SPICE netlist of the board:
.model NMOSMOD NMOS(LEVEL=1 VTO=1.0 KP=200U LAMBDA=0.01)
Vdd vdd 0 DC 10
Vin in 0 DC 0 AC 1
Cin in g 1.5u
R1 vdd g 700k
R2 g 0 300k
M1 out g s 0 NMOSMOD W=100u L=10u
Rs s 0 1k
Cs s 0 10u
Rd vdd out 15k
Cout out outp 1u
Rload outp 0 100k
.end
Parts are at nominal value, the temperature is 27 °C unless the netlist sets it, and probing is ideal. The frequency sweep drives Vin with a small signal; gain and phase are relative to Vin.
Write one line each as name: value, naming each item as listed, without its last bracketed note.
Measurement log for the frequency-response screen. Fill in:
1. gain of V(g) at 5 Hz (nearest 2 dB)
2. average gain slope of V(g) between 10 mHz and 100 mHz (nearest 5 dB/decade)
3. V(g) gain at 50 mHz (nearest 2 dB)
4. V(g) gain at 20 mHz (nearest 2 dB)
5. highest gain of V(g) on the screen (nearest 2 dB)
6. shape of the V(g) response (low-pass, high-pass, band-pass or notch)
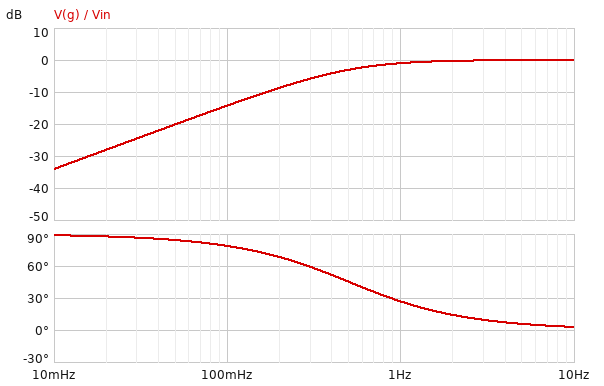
gain of V(g) at 5 Hz: 0 dB
average gain slope of V(g) between 10 mHz and 100 mHz: 20 dB/decade
V(g) gain at 50 mHz: -20 dB
V(g) gain at 20 mHz: -28 dB
highest gain of V(g) on the screen: 0 dB
shape of the V(g) response: high-pass
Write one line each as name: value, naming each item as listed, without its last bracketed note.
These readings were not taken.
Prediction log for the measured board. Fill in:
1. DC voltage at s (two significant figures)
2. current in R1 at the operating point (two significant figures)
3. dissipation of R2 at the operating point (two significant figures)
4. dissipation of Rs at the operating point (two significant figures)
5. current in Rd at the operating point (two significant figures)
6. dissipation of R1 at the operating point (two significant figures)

DC voltage at s: 610 mV
current in R1 at the operating point: 10 µA
dissipation of R2 at the operating point: 30 µW
dissipation of Rs at the operating point: 370 µW
current in Rd at the operating point: 610 µA
dissipation of R1 at the operating point: 70 µW
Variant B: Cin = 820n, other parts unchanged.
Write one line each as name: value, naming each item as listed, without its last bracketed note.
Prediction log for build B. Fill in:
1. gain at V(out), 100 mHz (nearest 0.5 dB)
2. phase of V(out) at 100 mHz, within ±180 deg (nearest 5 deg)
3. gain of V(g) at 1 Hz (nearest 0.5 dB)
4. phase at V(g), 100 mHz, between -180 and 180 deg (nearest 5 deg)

gain at V(out), 100 mHz: -34.0 dB
phase of V(out) at 100 mHz, within ±180 deg: -95 deg
gain of V(g) at 1 Hz: -2.5 dB
phase at V(g), 100 mHz, between -180 and 180 deg: 85 deg
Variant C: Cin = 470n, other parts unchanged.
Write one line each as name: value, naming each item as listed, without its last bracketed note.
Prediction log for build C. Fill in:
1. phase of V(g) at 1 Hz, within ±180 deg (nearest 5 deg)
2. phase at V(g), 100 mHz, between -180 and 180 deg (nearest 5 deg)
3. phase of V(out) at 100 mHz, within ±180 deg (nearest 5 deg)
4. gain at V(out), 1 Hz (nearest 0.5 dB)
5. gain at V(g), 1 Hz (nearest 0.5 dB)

phase of V(g) at 1 Hz, within ±180 deg: 60 deg
phase at V(g), 100 mHz, between -180 and 180 deg: 85 deg
phase of V(out) at 100 mHz, within ±180 deg: -95 deg
gain at V(out), 1 Hz: -20.0 dB
gain at V(g), 1 Hz: -5.5 dB
